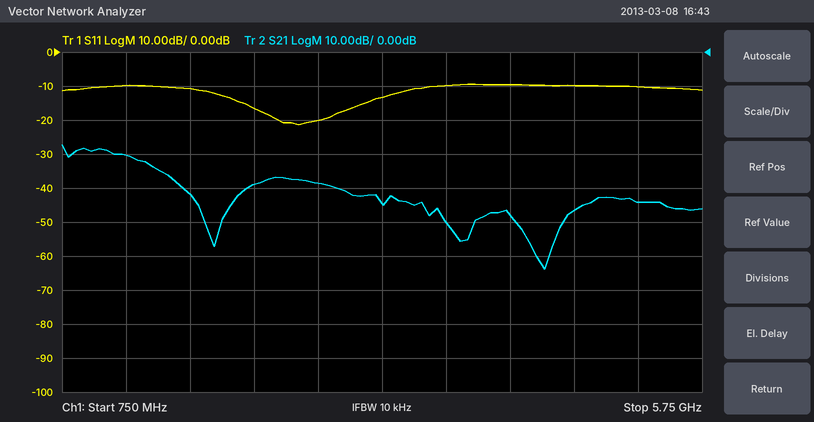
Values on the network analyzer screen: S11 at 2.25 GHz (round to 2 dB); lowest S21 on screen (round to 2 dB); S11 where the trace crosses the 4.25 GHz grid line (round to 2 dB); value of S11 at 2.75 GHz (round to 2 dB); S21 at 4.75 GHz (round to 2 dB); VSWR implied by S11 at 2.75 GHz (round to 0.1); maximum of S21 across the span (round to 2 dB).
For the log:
-16 dB
-64 dB
-10 dB
-20 dB
-46 dB
1.2
-28 dB
